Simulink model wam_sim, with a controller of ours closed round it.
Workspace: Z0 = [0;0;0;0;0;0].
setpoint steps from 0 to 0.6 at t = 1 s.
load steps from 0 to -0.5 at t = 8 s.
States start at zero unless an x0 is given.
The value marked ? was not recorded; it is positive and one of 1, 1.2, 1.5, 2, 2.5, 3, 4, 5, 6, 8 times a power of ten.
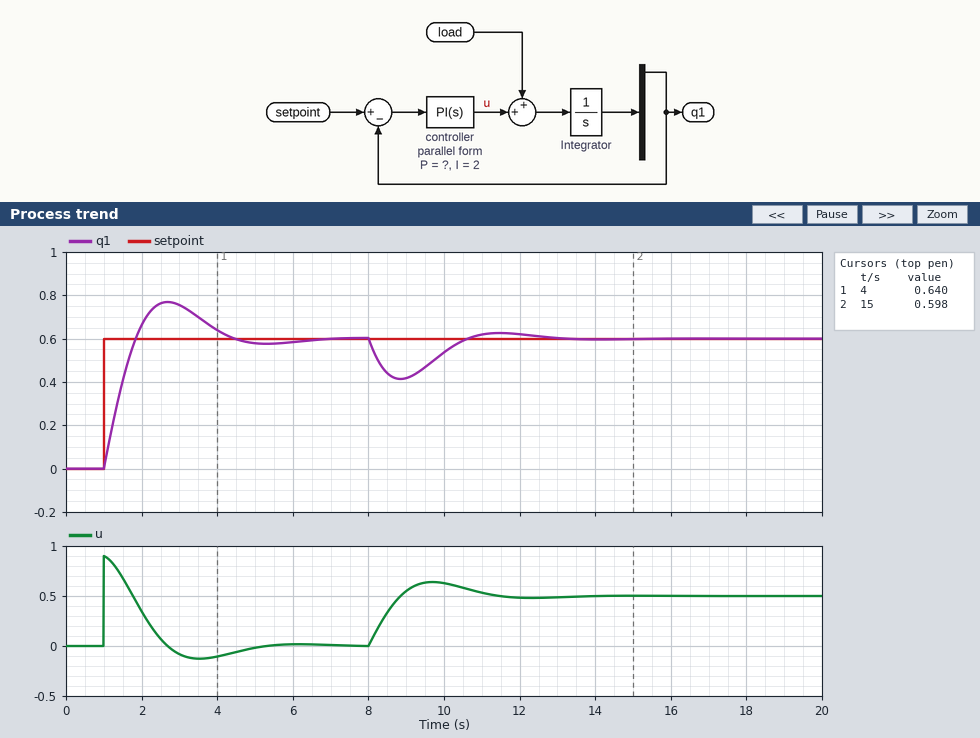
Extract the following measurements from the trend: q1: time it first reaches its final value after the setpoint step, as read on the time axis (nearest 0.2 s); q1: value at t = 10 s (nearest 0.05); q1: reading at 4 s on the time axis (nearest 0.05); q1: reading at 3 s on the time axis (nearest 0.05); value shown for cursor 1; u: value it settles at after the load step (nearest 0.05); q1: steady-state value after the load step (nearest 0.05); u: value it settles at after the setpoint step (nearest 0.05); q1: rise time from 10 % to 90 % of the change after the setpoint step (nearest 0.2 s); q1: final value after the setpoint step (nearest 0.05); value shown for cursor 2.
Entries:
1.8 s
0.55
0.65
0.75
0.640
0.50
0.60
0.00
0.6 s
0.60
0.598
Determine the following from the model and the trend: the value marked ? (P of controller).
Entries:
1.5
